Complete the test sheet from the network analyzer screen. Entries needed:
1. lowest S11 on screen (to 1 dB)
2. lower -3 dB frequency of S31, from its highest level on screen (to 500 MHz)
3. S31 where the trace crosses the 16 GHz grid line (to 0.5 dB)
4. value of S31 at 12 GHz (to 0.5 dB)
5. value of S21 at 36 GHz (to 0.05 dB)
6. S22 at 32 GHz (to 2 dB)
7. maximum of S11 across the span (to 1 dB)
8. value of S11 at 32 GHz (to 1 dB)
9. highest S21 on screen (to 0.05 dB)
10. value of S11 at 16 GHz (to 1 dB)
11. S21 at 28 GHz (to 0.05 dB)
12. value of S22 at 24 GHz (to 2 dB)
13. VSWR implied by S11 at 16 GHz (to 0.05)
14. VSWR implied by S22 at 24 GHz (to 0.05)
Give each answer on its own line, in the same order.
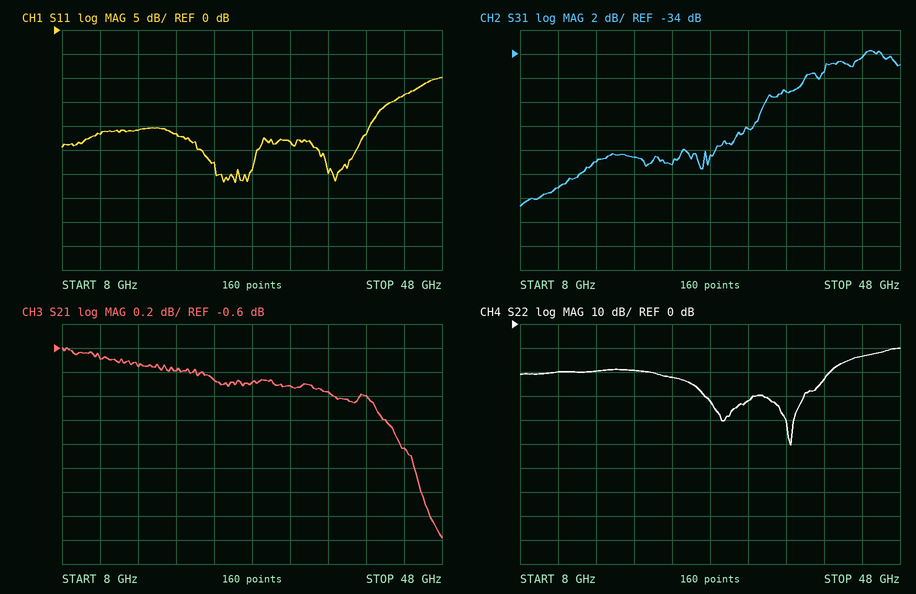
-32 dB
37.5 GHz
-43.0 dB
-45.0 dB
-0.95 dB
-32 dB
-10 dB
-23 dB
-0.60 dB
-21 dB
-0.90 dB
-22 dB
1.20
1.15
